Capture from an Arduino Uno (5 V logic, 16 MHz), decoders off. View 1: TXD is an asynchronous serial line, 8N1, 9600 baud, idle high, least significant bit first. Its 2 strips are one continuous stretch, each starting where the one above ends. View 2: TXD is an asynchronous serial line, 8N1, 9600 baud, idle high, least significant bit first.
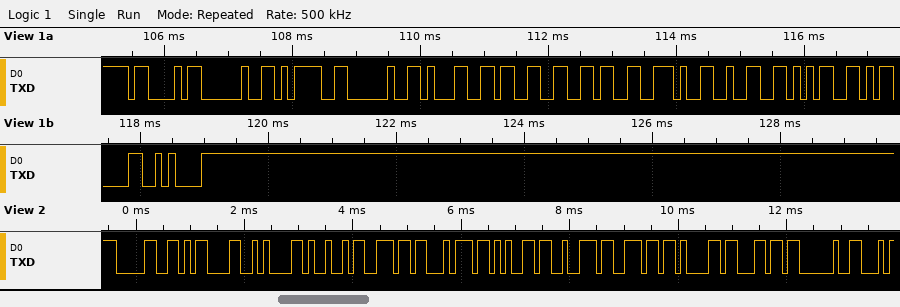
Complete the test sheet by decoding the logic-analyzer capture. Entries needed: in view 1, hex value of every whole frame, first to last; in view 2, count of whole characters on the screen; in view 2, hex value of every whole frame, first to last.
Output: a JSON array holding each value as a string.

["43 20 3D 20 31 33 36 2E 32 35 0D 0A", "12", "30 0D 0A 49 6E 74 65 72 6E 61 6C 20"]
